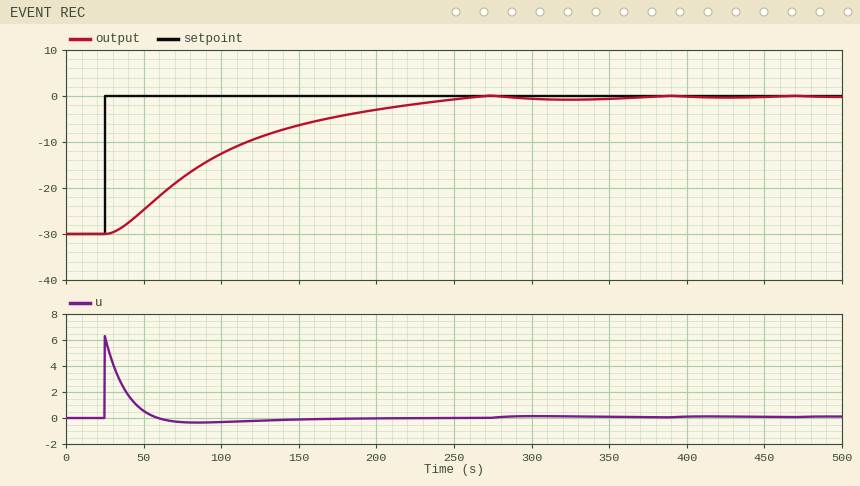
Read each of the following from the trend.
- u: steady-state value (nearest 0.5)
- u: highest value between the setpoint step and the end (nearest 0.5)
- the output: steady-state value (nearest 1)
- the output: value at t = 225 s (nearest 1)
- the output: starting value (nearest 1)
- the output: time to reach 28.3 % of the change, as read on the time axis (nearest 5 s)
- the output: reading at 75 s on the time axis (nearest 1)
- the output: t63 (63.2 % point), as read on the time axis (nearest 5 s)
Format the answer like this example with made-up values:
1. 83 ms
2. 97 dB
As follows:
1. 0.0
2. 6.5
3. 0
4. -2
5. -30
6. 60 s
7. -18
8. 110 s
